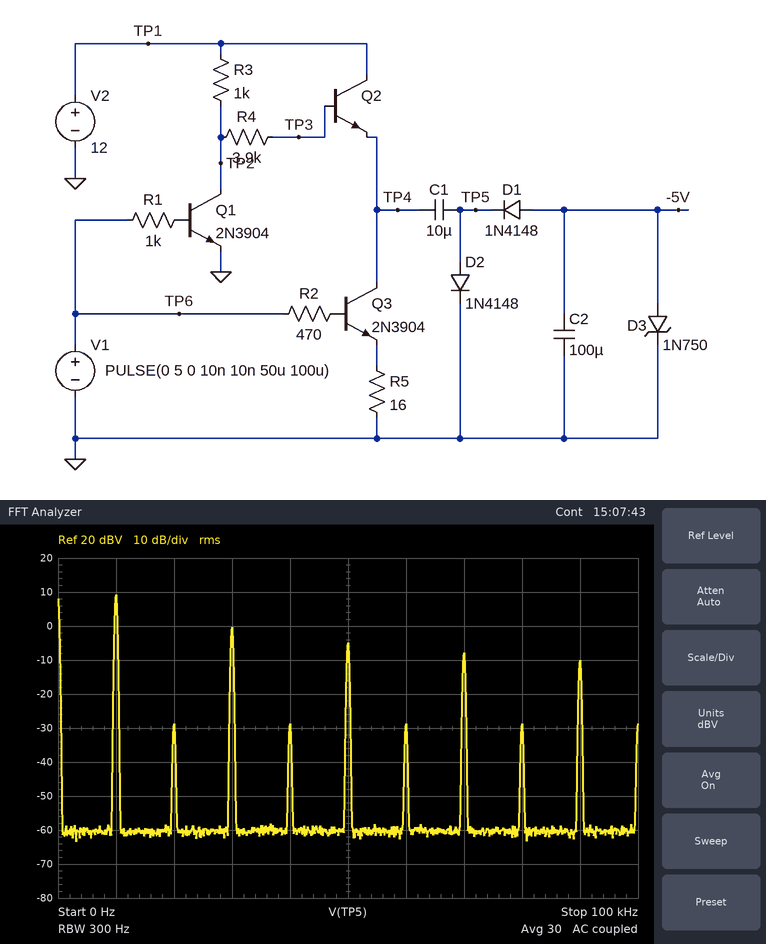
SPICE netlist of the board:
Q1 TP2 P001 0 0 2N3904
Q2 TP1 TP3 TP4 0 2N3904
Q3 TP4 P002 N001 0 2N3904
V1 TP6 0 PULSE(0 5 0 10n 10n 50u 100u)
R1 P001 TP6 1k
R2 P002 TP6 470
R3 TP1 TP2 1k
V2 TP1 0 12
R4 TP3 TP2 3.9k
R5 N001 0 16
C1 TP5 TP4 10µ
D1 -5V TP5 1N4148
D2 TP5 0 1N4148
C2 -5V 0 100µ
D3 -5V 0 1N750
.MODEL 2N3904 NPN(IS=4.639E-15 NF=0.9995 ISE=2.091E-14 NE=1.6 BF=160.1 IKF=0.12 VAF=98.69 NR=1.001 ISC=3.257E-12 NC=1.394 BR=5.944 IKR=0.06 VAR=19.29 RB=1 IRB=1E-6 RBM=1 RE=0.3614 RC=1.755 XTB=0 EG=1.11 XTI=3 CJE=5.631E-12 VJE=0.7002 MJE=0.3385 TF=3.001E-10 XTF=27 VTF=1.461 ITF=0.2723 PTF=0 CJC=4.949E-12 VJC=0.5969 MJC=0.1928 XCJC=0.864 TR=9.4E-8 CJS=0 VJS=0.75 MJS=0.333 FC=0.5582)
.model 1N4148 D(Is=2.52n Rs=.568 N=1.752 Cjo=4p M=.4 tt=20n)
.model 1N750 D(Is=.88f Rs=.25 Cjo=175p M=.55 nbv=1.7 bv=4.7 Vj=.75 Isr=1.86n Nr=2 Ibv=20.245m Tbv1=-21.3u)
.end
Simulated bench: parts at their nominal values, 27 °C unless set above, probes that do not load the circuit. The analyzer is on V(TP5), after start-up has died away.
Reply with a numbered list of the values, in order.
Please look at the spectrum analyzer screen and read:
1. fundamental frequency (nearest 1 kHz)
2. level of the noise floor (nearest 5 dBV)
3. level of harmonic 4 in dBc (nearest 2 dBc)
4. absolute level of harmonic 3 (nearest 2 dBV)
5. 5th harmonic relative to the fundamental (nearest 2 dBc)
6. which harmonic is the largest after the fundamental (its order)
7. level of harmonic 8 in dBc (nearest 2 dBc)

1. 10 kHz
2. -60 dBV
3. -38 dBc
4. 0 dBV
5. -14 dBc
6. 3
7. -38 dBc
